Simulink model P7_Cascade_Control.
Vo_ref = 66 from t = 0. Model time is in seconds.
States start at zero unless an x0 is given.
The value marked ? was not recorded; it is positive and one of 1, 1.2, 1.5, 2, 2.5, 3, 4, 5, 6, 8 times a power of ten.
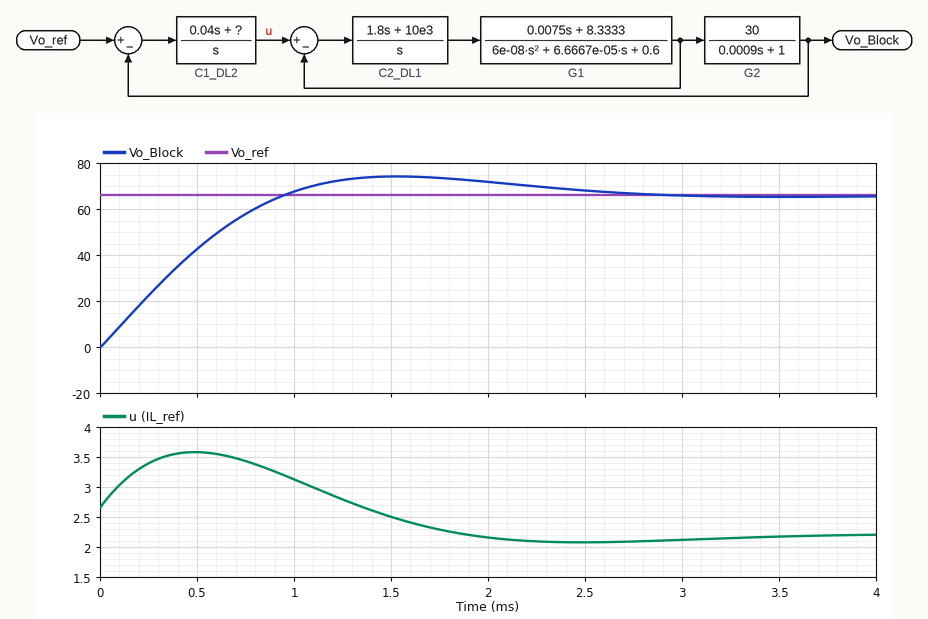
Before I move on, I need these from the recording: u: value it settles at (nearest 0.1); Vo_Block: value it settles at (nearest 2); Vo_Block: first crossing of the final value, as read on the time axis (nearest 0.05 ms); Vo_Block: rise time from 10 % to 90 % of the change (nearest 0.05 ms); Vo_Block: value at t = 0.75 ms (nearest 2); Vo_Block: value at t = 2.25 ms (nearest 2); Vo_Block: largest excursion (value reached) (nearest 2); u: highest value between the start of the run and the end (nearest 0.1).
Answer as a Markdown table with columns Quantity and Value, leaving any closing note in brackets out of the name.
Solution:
| Quantity | Value |
|---|---|
| u: value it settles at | 2.2 |
| Vo_Block: value it settles at | 66 |
| Vo_Block: first crossing of the final value, as read on the time axis | 0.95 ms |
| Vo_Block: rise time from 10 % to 90 % of the change | 0.70 ms |
| Vo_Block: value at t = 0.75 ms | 58 |
| Vo_Block: value at t = 2.25 ms | 70 |
| Vo_Block: largest excursion (value reached) | 74 |
| u: highest value between the start of the run and the end | 3.6 |
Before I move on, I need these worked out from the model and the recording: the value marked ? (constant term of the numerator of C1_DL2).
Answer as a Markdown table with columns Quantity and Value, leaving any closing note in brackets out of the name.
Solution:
| Quantity | Value |
|---|---|
| the value marked ? | 120 |
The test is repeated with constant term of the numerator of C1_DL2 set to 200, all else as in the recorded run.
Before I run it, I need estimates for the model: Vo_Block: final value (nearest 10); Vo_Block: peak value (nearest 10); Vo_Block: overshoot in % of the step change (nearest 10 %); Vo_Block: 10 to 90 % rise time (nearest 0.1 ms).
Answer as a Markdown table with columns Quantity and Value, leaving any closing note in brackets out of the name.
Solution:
| Quantity | Value |
|---|---|
| Vo_Block: final value | 70 |
| Vo_Block: peak value | 80 |
| Vo_Block: overshoot in % of the step change | 20 % |
| Vo_Block: 10 to 90 % rise time | 0.5 ms |
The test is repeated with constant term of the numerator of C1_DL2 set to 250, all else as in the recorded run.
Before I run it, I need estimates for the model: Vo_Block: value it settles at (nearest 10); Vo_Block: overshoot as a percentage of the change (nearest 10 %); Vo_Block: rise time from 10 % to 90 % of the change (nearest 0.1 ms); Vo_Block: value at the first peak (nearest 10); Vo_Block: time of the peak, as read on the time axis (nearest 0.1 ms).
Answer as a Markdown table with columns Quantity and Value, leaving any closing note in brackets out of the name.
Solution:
| Quantity | Value |
|---|---|
| Vo_Block: value it settles at | 70 |
| Vo_Block: overshoot as a percentage of the change | 30 % |
| Vo_Block: rise time from 10 % to 90 % of the change | 0.4 ms |
| Vo_Block: value at the first peak | 80 |
| Vo_Block: time of the peak, as read on the time axis | 1.0 ms |
